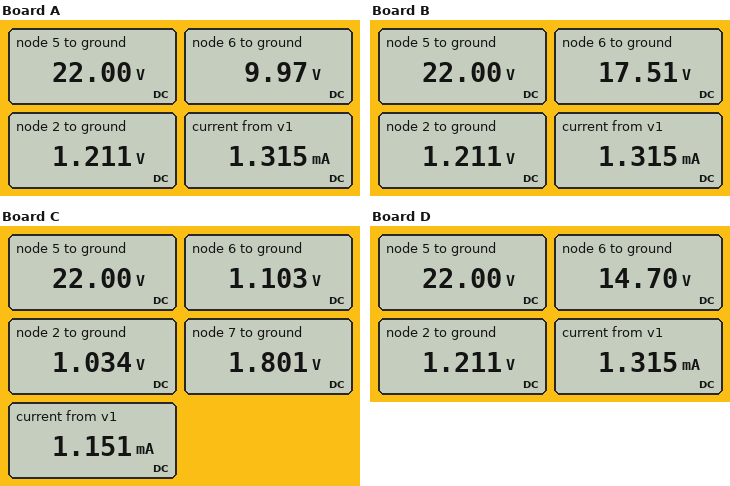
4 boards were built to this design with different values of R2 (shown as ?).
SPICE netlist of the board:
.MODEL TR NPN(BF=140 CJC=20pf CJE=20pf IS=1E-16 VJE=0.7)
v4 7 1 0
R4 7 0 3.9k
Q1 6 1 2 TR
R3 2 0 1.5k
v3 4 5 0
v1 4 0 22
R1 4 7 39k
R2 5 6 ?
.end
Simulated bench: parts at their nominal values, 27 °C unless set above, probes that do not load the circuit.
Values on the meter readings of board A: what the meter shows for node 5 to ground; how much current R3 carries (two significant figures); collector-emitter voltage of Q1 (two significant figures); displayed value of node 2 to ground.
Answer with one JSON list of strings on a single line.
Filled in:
["22.00 V", "810 µA", "8.8 V", "1.211 V"]
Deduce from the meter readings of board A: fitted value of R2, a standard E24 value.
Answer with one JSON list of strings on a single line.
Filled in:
["15 kΩ"]
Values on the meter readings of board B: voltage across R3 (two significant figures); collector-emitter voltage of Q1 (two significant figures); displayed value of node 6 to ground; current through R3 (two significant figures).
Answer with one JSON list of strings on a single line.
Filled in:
["1.2 V", "16 V", "17.51 V", "810 µA"]
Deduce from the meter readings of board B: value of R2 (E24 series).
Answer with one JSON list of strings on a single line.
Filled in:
["5.6 kΩ"]
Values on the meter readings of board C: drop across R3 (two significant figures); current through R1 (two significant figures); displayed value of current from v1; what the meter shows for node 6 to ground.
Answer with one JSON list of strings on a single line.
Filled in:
["1.0 V", "520 µA", "1.151 mA", "1.103 V"]
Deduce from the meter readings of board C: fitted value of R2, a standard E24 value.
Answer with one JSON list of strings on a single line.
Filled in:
["33 kΩ"]
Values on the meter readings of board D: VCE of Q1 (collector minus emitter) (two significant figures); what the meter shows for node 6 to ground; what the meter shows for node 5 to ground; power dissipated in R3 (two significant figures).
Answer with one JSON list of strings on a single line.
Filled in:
["13 V", "14.70 V", "22.00 V", "980 µW"]
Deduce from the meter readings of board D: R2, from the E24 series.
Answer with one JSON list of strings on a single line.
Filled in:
["9.1 kΩ"]
